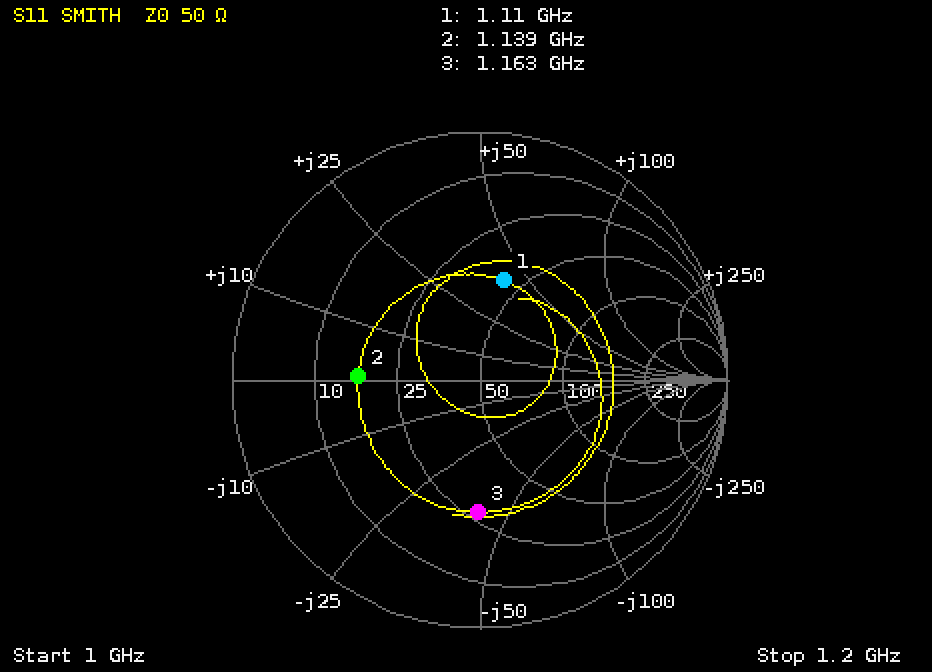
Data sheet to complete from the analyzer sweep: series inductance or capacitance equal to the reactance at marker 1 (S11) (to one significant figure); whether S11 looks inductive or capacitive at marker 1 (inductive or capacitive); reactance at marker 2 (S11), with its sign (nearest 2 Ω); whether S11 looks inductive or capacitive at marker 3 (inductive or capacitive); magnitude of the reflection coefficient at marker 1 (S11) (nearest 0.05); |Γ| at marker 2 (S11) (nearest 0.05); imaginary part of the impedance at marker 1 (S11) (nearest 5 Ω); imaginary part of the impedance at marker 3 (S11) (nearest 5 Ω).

6 nH
inductive
0 Ω
capacitive
0.40
0.50
+40 Ω
-40 Ω
